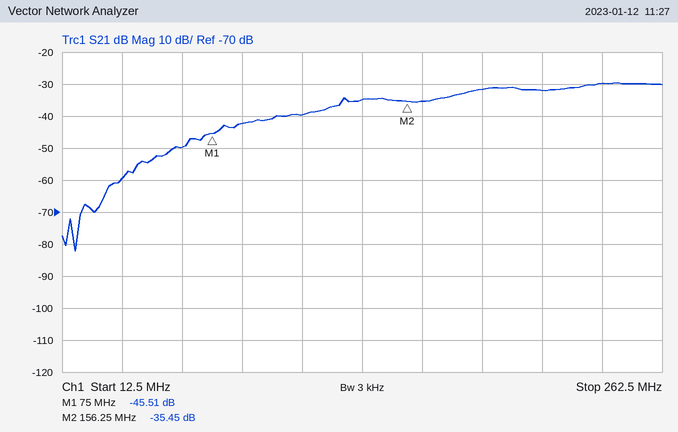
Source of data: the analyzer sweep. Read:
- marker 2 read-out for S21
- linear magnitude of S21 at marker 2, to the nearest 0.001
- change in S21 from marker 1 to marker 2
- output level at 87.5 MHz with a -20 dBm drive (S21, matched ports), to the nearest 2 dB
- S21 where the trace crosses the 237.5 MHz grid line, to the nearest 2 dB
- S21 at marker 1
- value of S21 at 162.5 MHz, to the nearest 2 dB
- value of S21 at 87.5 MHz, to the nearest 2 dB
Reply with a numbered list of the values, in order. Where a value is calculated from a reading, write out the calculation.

1. -35.45 dB
2. 10^(-35.45/20) ≈ 0.017
3. -35.45 − (-45.51) = 10.06 dB
4. -20 dBm + (-42 dB) = -62 dBm
5. -30 dB
6. -45.51 dB
7. -36 dB
8. -42 dB
